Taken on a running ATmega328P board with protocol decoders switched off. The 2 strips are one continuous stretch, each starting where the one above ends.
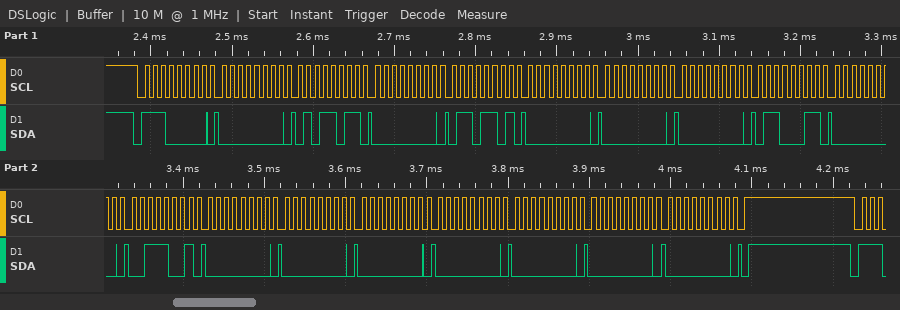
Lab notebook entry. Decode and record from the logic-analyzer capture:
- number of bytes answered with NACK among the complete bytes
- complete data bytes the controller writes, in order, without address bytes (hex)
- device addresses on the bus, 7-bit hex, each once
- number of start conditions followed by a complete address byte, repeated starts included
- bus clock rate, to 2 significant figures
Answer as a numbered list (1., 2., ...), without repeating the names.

1. 0
2. 00 5B 00 6D 00 00 00 63 00 39 00 00 00 00 00 00 00
3. 0x70
4. 1
5. 100 kHz
